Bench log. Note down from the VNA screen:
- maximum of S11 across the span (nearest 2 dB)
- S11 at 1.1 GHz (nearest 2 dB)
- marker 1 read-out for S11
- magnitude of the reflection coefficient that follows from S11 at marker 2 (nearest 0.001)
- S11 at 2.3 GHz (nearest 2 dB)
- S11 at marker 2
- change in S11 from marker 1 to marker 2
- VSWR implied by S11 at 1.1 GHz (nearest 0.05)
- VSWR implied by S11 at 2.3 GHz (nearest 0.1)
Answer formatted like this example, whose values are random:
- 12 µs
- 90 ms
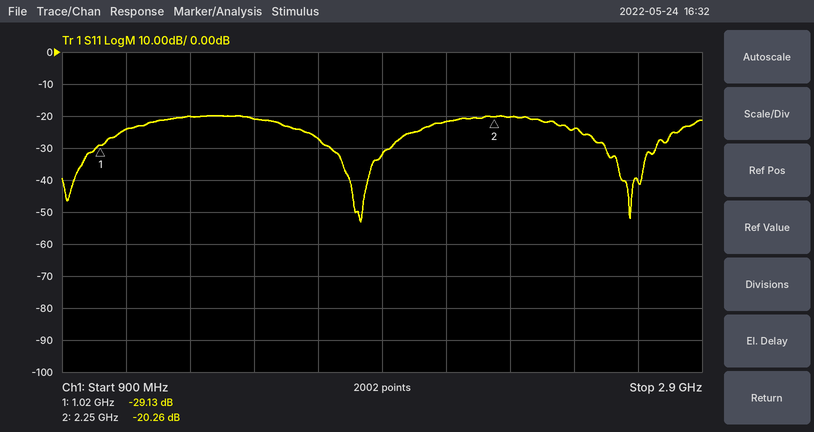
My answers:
- -20 dB
- -24 dB
- -29.13 dB
- 0.097
- -20 dB
- -20.26 dB
- 8.87 dB
- 1.15
- 1.2
